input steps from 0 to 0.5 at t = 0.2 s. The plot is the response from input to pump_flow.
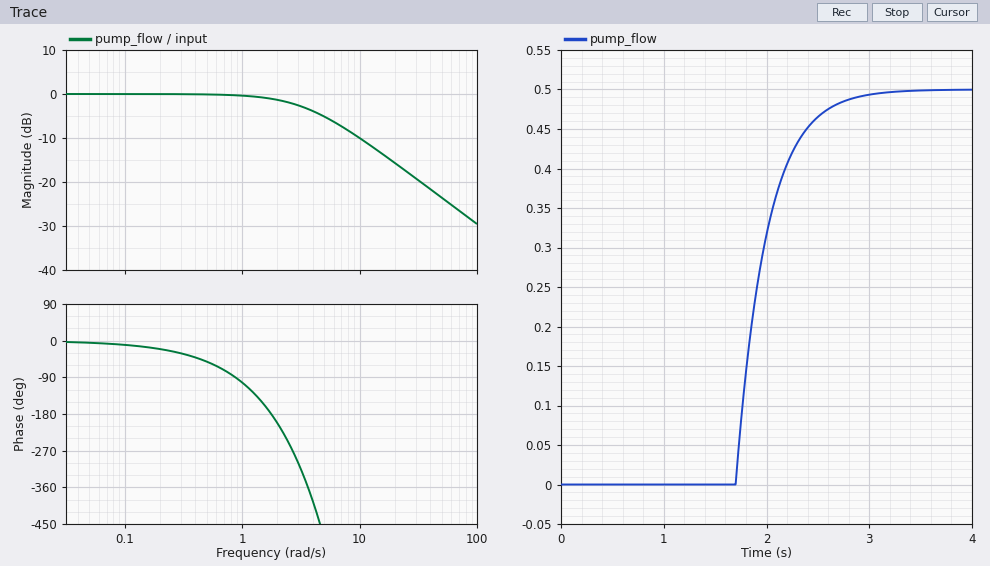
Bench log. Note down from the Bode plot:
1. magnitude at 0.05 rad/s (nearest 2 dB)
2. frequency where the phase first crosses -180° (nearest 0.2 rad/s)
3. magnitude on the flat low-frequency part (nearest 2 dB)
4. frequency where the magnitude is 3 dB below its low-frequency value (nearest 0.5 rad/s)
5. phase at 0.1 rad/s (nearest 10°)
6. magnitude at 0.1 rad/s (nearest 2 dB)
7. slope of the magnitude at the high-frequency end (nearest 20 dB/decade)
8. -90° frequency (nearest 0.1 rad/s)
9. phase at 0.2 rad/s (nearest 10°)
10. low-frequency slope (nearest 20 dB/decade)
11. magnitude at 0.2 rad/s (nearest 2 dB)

0 dB
1.8 rad/s
0 dB
3.5 rad/s
-10°
0 dB
-20 dB/decade
0.9 rad/s
-20°
0 dB/decade
0 dB
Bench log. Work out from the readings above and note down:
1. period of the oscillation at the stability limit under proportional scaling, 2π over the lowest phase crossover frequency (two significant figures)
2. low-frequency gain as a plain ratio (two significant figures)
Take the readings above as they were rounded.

3.5 s
1.0
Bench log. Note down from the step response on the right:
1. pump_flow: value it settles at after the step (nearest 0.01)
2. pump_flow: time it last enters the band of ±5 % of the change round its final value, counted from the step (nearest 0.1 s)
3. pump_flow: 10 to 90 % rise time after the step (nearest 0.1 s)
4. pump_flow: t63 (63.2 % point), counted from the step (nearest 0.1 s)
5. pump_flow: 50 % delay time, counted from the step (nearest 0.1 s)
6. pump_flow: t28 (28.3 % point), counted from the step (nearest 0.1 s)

0.50
2.4 s
0.7 s
1.8 s
1.7 s
1.6 s
